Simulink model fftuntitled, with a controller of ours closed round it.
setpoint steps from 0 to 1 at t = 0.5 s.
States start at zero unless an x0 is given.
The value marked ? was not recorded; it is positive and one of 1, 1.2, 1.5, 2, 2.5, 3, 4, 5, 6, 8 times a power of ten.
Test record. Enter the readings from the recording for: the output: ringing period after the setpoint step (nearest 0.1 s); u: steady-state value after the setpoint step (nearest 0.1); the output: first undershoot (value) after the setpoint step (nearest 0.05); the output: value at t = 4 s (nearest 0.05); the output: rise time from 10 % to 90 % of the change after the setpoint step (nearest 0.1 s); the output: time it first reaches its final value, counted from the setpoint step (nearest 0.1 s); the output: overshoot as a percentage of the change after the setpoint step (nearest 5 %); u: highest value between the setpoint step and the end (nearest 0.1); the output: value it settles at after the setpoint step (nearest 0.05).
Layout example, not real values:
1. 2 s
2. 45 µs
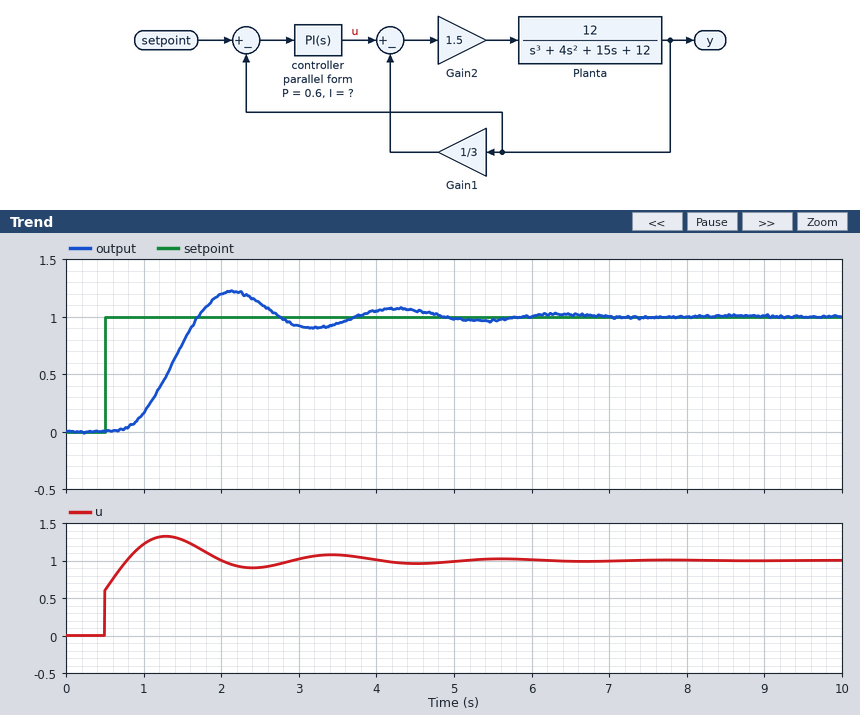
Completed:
1. 2.1 s
2. 1.0
3. 0.90
4. 1.05
5. 0.7 s
6. 1.2 s
7. 20 %
8. 1.3
9. 1.00
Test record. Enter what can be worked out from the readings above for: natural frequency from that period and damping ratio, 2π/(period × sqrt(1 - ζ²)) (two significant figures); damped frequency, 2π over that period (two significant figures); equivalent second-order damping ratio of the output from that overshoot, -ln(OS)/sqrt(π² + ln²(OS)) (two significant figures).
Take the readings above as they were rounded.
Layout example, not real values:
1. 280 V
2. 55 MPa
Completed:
1. 3.4 rad/s
2. 3.0 rad/s
3. 0.46
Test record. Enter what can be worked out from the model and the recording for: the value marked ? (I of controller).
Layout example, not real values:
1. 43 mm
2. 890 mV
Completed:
1. 1.5
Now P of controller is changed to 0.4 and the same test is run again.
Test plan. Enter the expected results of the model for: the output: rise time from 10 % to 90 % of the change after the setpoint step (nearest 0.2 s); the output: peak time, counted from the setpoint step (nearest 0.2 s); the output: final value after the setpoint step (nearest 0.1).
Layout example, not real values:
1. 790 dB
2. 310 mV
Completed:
1. 0.8 s
2. 1.8 s
3. 1.0
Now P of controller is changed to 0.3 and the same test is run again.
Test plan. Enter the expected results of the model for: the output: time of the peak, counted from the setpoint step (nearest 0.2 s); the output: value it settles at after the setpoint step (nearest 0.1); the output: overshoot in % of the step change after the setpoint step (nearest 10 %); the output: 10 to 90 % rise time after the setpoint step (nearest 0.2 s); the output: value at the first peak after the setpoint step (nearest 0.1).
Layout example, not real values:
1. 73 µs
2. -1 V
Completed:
1. 2.0 s
2. 1.0
3. 30 %
4. 0.8 s
5. 1.3
